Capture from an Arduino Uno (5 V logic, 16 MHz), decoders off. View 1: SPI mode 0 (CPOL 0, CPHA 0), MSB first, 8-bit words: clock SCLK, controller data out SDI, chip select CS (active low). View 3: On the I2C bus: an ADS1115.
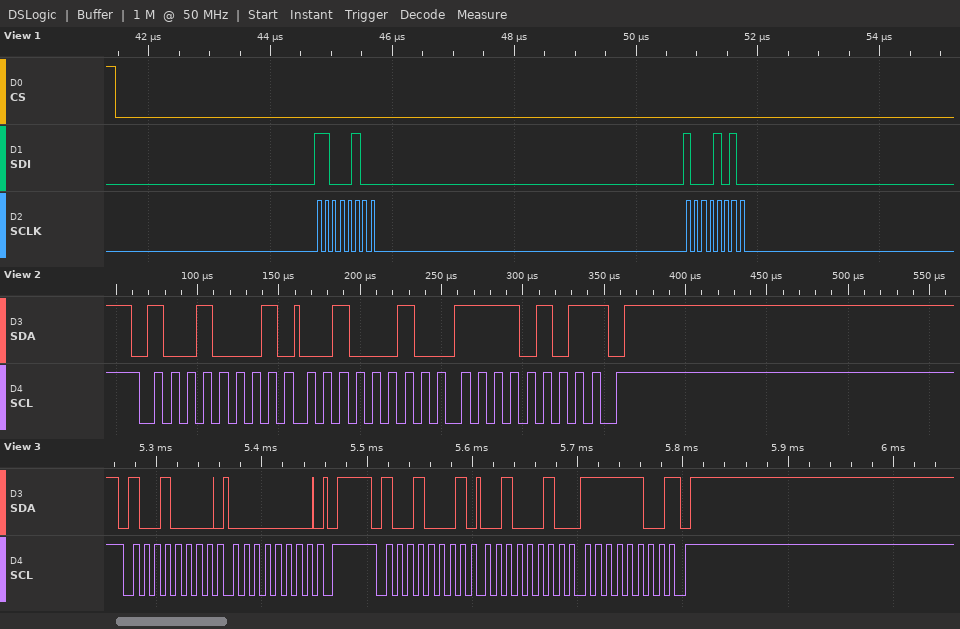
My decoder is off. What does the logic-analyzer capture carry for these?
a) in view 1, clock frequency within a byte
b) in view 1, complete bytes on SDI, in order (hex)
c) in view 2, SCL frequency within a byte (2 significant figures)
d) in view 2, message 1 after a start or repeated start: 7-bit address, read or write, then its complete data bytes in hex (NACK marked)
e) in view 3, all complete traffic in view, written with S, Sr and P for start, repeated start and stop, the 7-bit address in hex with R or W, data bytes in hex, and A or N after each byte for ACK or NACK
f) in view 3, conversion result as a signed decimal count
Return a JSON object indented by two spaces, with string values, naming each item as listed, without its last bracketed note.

{
  "in view 1, clock frequency within a byte": "8 MHz",
  "in view 1, complete bytes on SDI, in order": "0xC4 0x8A",
  "in view 2, SCL frequency within a byte": "100 kHz",
  "in view 2, message 1 after a start or repeated start: 7-bit address, read or write, then its complete data bytes in hex": "0x48 read: 22 F5 NACK",
  "in view 3, all complete traffic in view, written with S, Sr and P for start, repeated start and stop, the 7-bit address in hex with R or W, data bytes in hex, and A or N after each byte for ACK or NACK": "S 48W A 00 A P S 48R A 22 A FC N P",
  "in view 3, conversion result as a signed decimal count": "8956"
}
